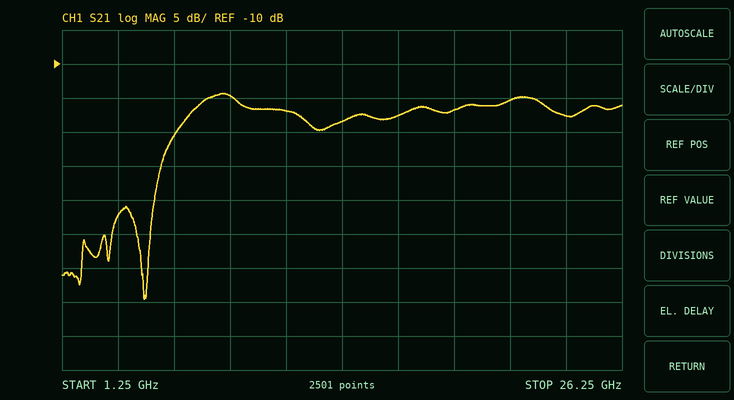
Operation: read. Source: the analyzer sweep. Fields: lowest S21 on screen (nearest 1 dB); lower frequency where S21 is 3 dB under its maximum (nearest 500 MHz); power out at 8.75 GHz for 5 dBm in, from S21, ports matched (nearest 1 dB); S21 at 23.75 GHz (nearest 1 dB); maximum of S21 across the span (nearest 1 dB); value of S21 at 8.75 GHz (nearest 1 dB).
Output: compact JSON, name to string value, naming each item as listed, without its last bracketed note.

{"lowest S21 on screen": "-45 dB", "lower frequency where S21 is 3 dB under its maximum": "7.0 GHz", "power out at 8.75 GHz for 5 dBm in, from S21, ports matched": "-10 dBm", "S21 at 23.75 GHz": "-18 dB", "maximum of S21 across the span": "-14 dB", "value of S21 at 8.75 GHz": "-15 dB"}
